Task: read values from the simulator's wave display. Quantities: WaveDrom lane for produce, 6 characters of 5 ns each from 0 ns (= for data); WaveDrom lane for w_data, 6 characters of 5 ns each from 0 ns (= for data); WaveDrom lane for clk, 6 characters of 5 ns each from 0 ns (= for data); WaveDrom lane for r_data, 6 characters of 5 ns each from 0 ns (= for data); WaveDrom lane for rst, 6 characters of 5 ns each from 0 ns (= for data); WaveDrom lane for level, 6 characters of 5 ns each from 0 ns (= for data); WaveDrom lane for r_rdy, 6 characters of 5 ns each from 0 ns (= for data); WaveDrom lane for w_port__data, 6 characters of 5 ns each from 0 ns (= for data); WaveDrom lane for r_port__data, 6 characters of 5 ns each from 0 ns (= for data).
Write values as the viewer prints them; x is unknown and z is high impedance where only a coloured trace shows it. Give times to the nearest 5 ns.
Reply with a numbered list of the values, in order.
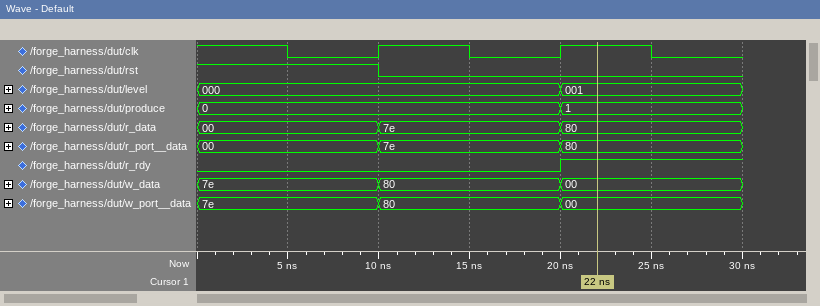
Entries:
1. {name: 'produce', wave: '=...=.', data: '0 1'}
2. {name: 'w_data', wave: '=.=.=.', data: '7e 80 00'}
3. {name: 'clk', wave: '101010'}
4. {name: 'r_data', wave: '=.=.=.', data: '00 7e 80'}
5. {name: 'rst', wave: '1.0...'}
6. {name: 'level', wave: '=...=.', data: '000 001'}
7. {name: 'r_rdy', wave: '0...1.'}
8. {name: 'w_port__data', wave: '=.=.=.', data: '7e 80 00'}
9. {name: 'r_port__data', wave: '=.=.=.', data: '00 7e 80'}
